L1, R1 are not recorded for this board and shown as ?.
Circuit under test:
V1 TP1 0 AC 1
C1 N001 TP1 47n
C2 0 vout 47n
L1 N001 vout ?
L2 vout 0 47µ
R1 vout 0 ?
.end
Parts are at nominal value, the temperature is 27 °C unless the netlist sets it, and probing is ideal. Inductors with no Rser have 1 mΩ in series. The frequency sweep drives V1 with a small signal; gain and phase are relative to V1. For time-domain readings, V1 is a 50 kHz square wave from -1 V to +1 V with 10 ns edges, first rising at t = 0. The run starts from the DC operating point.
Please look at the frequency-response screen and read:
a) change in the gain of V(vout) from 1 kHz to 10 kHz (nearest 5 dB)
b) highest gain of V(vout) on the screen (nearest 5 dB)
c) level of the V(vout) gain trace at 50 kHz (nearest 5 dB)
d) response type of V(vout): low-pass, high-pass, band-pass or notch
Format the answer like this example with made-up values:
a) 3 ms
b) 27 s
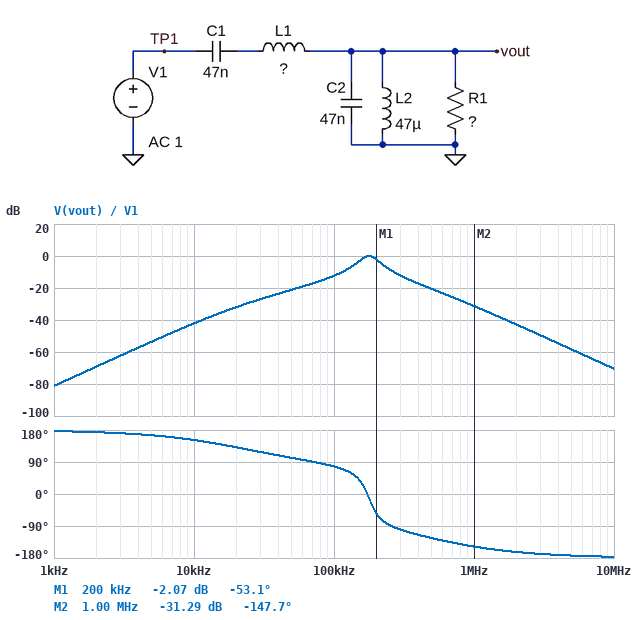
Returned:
a) 40 dB
b) 0 dB
c) -20 dB
d) band-pass
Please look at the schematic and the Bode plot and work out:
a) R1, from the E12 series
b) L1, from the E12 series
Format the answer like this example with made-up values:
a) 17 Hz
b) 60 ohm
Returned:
a) 5.6 Ω
b) 18 µH
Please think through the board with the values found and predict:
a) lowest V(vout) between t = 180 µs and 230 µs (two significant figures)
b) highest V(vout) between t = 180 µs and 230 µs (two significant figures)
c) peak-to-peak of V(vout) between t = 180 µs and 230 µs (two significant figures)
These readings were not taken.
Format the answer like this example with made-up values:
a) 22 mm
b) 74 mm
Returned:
a) -450 mV
b) 450 mV
c) 890 mV
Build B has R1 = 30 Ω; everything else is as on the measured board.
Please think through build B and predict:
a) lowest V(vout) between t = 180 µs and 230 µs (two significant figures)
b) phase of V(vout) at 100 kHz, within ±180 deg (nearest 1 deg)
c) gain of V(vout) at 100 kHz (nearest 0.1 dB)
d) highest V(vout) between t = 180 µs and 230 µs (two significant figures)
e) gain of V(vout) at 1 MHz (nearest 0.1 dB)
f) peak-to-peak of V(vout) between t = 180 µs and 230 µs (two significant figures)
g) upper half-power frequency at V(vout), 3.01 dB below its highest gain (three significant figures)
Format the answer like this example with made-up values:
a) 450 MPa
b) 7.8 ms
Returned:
a) -1.0 V
b) 40 deg
c) -1.4 dB
d) 1.0 V
e) -29.9 dB
f) 2.1 V
g) 276 kHz
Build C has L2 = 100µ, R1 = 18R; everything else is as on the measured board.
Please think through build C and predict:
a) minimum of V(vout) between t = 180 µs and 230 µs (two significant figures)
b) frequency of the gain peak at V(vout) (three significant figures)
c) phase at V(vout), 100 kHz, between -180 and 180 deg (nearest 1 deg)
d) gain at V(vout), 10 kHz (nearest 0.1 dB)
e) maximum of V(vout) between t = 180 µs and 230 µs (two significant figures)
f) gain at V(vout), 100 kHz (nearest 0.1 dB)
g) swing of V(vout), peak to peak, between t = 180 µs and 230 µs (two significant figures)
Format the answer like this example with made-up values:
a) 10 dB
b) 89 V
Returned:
a) -1.0 V
b) 223 kHz
c) 44 deg
d) -34.8 dB
e) 1.0 V
f) -5.2 dB
g) 2.0 V
